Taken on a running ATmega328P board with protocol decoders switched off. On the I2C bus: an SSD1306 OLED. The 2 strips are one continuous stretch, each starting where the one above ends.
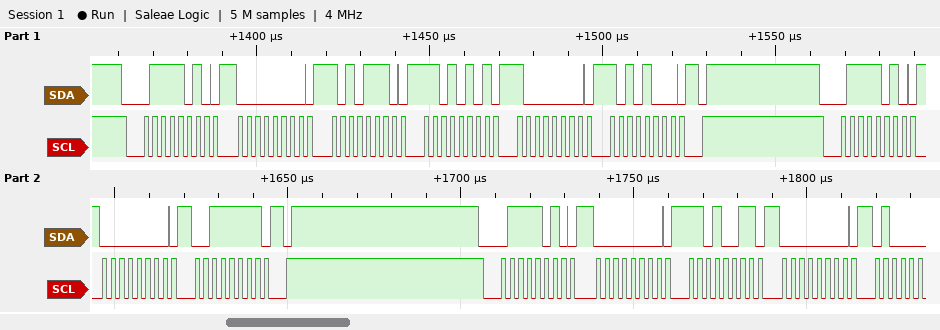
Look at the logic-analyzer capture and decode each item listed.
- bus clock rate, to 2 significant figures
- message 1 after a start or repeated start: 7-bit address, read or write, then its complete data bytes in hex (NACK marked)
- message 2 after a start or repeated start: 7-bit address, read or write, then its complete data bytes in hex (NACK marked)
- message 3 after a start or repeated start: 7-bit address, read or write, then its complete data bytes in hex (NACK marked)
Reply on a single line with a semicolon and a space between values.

400 kHz; 0x3D write: 00 AE D5 80 A8; 0x3D write: 00 3F; 0x3D write: 00 D3 00
